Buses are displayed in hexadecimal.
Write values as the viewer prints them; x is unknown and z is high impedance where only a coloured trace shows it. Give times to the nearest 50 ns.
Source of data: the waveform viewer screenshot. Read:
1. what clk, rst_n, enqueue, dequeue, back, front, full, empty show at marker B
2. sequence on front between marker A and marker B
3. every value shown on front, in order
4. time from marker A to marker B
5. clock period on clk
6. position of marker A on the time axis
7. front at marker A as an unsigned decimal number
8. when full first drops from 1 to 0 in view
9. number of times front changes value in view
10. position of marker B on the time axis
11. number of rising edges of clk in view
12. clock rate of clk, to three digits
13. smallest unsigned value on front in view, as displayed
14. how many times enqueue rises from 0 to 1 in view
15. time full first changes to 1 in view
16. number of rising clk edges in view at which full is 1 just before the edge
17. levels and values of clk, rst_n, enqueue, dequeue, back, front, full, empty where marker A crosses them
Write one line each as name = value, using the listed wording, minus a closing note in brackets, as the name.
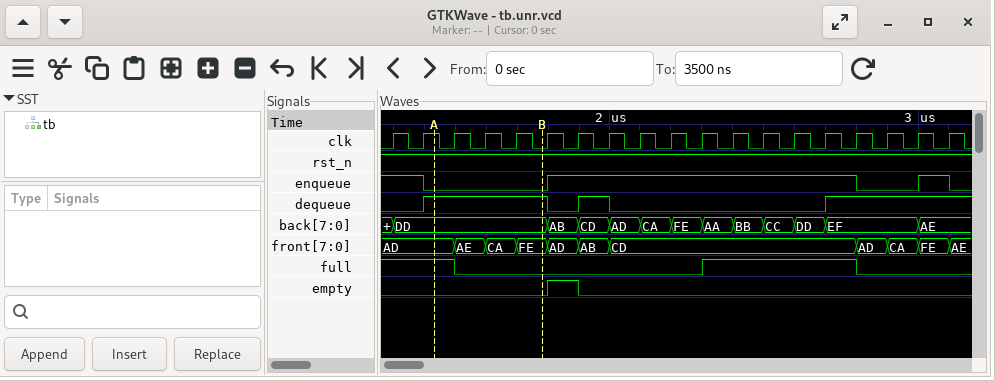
what clk, rst_n, enqueue, dequeue, back, front, full, empty show at marker B = clk=0, rst_n=1, enqueue=0, dequeue=1, back=DD, front=FE, full=0, empty=0
sequence on front between marker A and marker B = AD, AE, CA, FE
every value shown on front, in order = AD, AE, CA, FE, AD, AB, CD, AD, CA, FE, AE
time from marker A to marker B = 350 ns
clock period on clk = 100 ns
position of marker A on the time axis = 1450 ns
front at marker A as an unsigned decimal number = 173
when full first drops from 1 to 0 in view = 1500 ns
number of times front changes value in view = 10
position of marker B on the time axis = 1800 ns
number of rising edges of clk in view = 19
clock rate of clk, to three digits = 10.0 MHz
smallest unsigned value on front in view, as displayed = AB
how many times enqueue rises from 0 to 1 in view = 2
time full first changes to 1 in view = 2300 ns
number of rising clk edges in view at which full is 1 just before the edge = 8
levels and values of clk, rst_n, enqueue, dequeue, back, front, full, empty where marker A crosses them = clk=1, rst_n=1, enqueue=0, dequeue=1, back=DD, front=AD, full=1, empty=0
